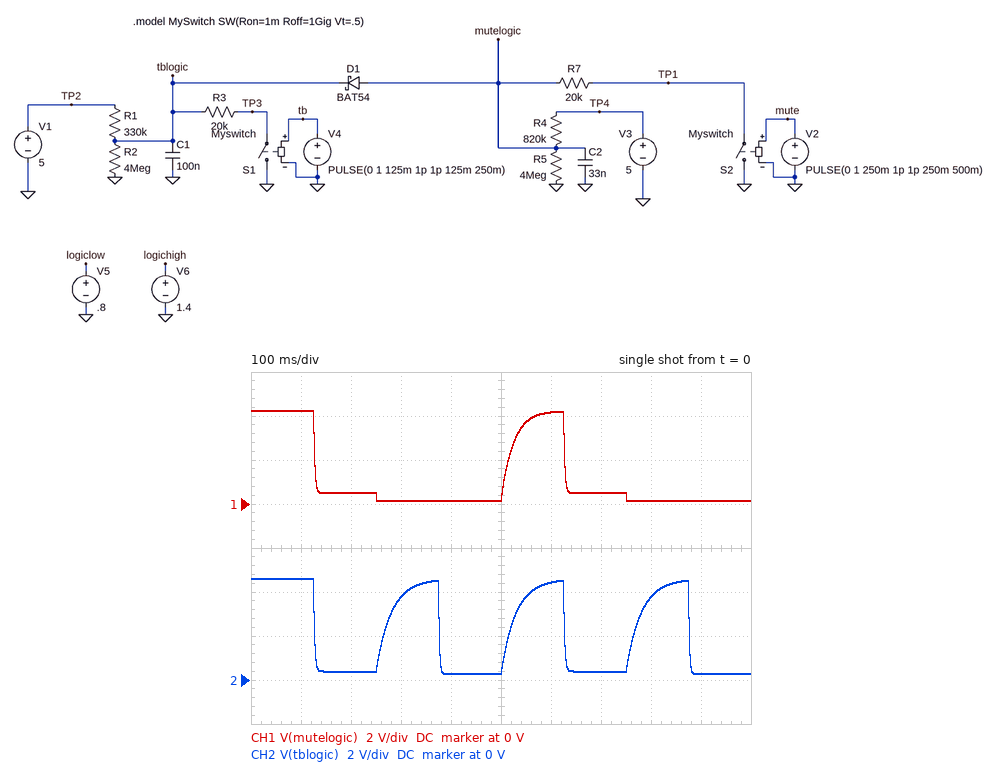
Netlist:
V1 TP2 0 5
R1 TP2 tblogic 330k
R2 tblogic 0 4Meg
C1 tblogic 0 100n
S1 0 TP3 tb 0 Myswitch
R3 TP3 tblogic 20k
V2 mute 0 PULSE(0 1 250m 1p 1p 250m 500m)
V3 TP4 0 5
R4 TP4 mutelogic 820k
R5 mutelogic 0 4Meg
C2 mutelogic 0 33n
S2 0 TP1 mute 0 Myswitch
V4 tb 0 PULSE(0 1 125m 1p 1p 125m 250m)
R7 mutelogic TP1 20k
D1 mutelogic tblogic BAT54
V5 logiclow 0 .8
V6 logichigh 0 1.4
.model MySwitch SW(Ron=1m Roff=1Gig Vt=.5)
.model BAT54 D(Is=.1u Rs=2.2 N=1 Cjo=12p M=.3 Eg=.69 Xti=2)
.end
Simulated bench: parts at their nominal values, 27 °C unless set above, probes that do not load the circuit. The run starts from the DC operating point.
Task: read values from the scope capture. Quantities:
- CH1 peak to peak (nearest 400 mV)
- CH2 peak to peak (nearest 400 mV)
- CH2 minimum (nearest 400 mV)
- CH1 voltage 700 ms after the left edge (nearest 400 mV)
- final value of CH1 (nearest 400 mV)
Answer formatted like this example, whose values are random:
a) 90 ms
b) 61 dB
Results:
a) 4.0 V
b) 4.4 V
c) 400 mV
d) 400 mV
e) 0 V
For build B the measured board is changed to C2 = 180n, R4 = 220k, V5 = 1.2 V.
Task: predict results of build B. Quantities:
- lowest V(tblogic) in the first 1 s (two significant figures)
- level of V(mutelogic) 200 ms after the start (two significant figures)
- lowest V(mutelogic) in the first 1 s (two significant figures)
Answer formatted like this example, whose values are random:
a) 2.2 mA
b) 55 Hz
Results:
a) 310 mV
b) 780 mV
c) 390 mV
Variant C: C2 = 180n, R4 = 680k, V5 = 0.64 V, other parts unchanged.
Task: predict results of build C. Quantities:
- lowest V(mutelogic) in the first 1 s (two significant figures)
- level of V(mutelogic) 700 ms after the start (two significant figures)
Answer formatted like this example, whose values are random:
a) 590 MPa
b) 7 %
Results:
a) 140 mV
b) 510 mV
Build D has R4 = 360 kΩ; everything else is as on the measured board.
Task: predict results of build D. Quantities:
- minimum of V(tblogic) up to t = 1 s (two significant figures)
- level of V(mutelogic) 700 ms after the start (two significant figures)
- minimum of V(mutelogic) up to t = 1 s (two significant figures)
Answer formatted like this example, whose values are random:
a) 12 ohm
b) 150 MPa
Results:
a) 280 mV
b) 630 mV
c) 260 mV
